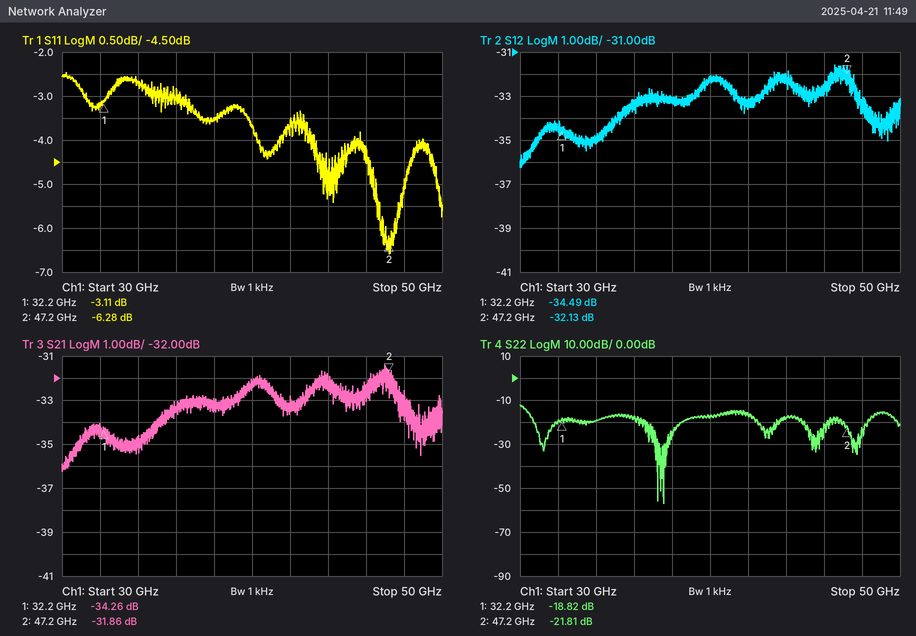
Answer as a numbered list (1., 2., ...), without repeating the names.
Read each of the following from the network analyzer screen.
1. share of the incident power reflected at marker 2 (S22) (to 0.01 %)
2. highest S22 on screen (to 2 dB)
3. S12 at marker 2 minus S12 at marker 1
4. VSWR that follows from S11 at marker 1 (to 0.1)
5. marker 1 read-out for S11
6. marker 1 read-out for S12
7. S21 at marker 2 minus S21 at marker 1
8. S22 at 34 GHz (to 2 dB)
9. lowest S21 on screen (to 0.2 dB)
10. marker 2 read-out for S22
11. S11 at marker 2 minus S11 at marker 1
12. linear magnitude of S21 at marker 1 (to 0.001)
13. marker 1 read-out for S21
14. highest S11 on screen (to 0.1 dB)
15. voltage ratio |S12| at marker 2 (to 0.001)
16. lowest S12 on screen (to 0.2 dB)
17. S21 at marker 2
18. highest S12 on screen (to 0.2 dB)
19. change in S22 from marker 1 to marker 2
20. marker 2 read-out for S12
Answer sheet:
1. 0.66 %
2. -12 dB
3. 2.36 dB
4. 5.6
5. -3.11 dB
6. -34.49 dB
7. 2.40 dB
8. -20 dB
9. -36.2 dB
10. -21.81 dB
11. -3.17 dB
12. 0.019
13. -34.26 dB
14. -2.5 dB
15. 0.025
16. -36.2 dB
17. -31.86 dB
18. -31.6 dB
19. -2.99 dB
20. -32.13 dB
